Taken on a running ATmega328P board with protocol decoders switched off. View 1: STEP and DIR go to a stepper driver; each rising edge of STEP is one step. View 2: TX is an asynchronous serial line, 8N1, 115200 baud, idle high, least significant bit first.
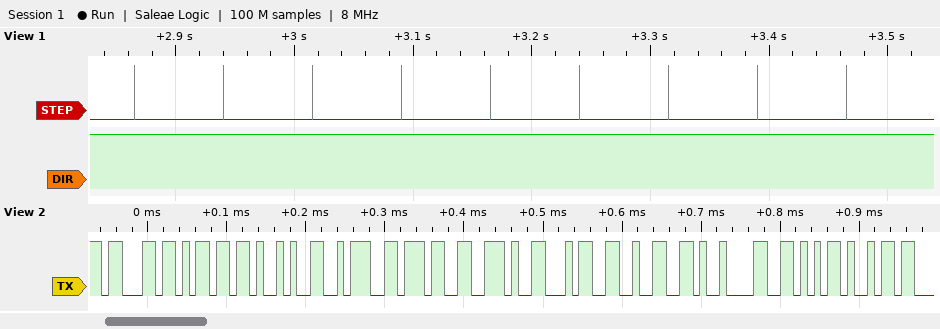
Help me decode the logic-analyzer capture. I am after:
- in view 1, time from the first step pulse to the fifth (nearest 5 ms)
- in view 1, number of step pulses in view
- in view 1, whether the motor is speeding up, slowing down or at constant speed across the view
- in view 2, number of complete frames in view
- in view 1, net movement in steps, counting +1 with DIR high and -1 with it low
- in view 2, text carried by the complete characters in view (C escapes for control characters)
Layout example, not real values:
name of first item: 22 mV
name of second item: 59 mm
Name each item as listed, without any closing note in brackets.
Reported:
in view 1, time from the first step pulse to the fifth: 300 ms
in view 1, number of step pulses in view: 9
in view 1, whether the motor is speeding up, slowing down or at constant speed across the view: constant speed
in view 2, number of complete frames in view: 11
in view 1, net movement in steps, counting +1 with DIR high and -1 with it low: +9
in view 2, text carried by the complete characters in view: "cm):7.42\tVi"
